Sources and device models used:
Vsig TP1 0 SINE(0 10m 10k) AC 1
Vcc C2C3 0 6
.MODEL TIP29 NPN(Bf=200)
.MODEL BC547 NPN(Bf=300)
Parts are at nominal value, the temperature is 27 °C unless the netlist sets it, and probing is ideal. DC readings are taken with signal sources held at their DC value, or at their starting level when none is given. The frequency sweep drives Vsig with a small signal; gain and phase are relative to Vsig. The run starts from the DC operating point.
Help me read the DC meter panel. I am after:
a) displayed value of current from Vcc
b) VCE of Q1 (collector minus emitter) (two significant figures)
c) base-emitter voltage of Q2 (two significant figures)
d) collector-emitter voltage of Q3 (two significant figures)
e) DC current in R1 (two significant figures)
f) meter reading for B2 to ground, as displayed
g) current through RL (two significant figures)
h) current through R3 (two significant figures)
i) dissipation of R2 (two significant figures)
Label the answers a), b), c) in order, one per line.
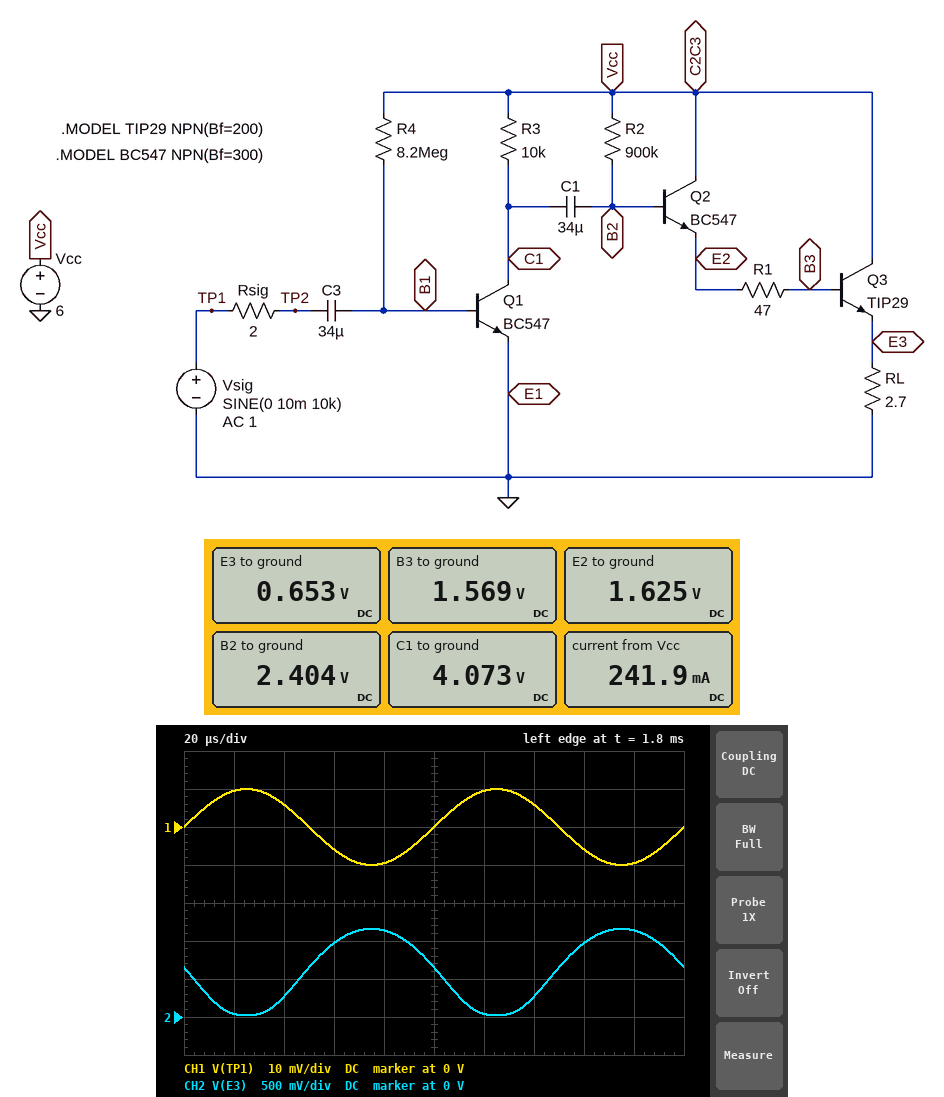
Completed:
a) 241.9 mA
b) 4.1 V
c) 780 mV
d) 5.3 V
e) 1.2 mA
f) 2.404 V
g) 240 mA
h) 190 µA
i) 14 µW
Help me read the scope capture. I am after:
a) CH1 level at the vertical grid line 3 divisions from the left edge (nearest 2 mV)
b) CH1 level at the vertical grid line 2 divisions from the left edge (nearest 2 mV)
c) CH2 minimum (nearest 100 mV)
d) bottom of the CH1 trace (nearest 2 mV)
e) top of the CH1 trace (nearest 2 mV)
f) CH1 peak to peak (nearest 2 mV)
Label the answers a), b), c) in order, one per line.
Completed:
a) -6 mV
b) 6 mV
c) 0 V
d) -10 mV
e) 10 mV
f) 20 mV
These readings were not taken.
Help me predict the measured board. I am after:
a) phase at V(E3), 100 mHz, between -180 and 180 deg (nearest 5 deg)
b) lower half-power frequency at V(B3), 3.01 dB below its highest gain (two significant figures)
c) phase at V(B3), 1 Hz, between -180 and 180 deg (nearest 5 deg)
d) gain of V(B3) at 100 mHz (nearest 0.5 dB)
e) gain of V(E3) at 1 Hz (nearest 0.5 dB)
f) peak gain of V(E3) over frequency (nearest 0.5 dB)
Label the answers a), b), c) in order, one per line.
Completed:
a) -115 deg
b) 120 mHz
c) -170 deg
d) 32.0 dB
e) 35.5 dB
f) 35.5 dB
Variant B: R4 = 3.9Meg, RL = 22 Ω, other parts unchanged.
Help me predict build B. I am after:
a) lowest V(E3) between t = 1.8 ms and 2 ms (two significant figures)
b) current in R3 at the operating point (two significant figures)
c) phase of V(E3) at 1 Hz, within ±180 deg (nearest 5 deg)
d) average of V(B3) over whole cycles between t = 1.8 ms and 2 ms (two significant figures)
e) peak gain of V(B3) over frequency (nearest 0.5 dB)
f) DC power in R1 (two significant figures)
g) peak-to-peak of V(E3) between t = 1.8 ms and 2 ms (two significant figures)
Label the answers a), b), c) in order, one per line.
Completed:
a) 830 mV
b) 400 µA
c) -165 deg
d) 3.3 V
e) 43.5 dB
f) 16 µW
g) 3.0 V
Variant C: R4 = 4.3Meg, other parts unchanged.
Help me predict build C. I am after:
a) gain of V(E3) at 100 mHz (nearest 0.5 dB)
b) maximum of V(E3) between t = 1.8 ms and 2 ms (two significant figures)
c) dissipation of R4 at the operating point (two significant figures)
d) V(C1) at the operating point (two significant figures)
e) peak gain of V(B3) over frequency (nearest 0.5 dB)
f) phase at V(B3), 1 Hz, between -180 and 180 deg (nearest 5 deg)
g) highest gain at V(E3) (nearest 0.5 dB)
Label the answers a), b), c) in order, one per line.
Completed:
a) 33.0 dB
b) 1.6 V
c) 6.4 µW
d) 2.3 V
e) 41.5 dB
f) -165 deg
g) 41.0 dB
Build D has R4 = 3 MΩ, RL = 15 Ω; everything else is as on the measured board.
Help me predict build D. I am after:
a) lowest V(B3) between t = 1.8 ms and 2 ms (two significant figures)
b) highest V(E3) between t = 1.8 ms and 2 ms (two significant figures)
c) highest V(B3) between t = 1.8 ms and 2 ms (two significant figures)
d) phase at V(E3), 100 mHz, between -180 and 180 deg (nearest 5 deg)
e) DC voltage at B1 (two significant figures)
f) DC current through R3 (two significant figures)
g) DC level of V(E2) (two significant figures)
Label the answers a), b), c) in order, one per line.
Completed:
a) 2.4 V
b) 3.9 V
c) 4.8 V
d) -100 deg
e) 760 mV
f) 520 µA
g) 3.1 V
